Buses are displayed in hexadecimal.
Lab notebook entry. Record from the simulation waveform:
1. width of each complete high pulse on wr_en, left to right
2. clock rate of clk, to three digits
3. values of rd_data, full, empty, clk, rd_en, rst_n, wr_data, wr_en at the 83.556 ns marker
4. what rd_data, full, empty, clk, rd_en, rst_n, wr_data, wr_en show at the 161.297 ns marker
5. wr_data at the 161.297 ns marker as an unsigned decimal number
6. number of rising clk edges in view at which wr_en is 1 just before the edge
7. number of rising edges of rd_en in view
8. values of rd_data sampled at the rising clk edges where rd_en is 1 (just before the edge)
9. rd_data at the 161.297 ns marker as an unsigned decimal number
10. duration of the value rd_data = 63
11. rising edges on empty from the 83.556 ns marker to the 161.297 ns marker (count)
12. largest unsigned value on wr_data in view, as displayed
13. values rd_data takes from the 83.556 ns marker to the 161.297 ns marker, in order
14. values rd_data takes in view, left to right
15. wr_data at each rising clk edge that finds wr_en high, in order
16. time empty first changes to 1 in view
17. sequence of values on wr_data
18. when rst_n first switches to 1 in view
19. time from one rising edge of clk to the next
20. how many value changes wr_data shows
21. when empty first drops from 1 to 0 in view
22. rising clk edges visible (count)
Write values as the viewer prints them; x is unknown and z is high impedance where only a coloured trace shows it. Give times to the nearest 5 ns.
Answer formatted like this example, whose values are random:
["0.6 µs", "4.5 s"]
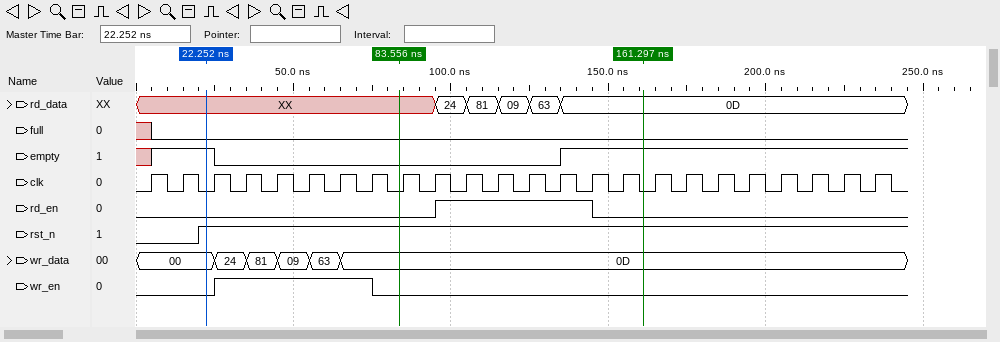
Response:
["50 ns", "100 MHz", "rd_data=XX, full=0, empty=0, clk=0, rd_en=0, rst_n=1, wr_data=0D, wr_en=0", "rd_data=0D, full=0, empty=1, clk=0, rd_en=0, rst_n=1, wr_data=0D, wr_en=0", "13", "5", "1", "24, 81, 09, 63, 0D", "13", "10 ns", "1", "81", "XX, 24, 81, 09, 63, 0D", "XX, 24, 81, 09, 63, 0D", "24, 81, 09, 63, 0D", "5 ns", "00, 24, 81, 09, 63, 0D", "20 ns", "10 ns", "5", "25 ns", "24"]
